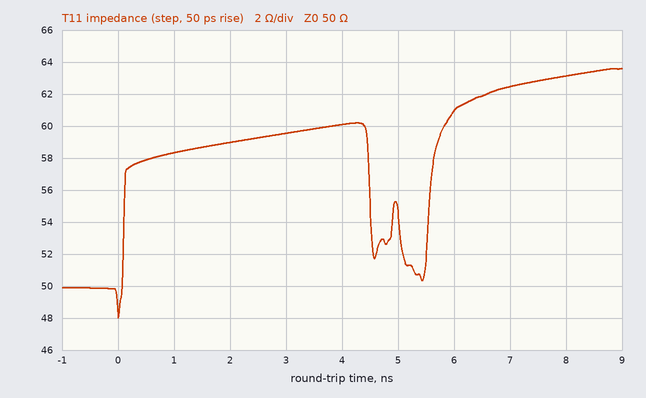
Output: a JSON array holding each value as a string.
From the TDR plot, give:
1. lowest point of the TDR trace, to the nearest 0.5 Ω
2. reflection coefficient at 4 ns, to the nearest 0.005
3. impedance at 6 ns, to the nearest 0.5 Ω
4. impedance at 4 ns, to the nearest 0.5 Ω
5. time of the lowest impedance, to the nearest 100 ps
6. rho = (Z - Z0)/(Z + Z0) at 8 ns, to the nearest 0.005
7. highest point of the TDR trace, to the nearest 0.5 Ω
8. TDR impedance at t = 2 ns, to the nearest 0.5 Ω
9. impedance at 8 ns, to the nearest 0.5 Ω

["48.0 Ω", "+0.090", "61.0 Ω", "60.0 Ω", "0.0 ns", "+0.115", "63.5 Ω", "59.0 Ω", "63.0 Ω"]
